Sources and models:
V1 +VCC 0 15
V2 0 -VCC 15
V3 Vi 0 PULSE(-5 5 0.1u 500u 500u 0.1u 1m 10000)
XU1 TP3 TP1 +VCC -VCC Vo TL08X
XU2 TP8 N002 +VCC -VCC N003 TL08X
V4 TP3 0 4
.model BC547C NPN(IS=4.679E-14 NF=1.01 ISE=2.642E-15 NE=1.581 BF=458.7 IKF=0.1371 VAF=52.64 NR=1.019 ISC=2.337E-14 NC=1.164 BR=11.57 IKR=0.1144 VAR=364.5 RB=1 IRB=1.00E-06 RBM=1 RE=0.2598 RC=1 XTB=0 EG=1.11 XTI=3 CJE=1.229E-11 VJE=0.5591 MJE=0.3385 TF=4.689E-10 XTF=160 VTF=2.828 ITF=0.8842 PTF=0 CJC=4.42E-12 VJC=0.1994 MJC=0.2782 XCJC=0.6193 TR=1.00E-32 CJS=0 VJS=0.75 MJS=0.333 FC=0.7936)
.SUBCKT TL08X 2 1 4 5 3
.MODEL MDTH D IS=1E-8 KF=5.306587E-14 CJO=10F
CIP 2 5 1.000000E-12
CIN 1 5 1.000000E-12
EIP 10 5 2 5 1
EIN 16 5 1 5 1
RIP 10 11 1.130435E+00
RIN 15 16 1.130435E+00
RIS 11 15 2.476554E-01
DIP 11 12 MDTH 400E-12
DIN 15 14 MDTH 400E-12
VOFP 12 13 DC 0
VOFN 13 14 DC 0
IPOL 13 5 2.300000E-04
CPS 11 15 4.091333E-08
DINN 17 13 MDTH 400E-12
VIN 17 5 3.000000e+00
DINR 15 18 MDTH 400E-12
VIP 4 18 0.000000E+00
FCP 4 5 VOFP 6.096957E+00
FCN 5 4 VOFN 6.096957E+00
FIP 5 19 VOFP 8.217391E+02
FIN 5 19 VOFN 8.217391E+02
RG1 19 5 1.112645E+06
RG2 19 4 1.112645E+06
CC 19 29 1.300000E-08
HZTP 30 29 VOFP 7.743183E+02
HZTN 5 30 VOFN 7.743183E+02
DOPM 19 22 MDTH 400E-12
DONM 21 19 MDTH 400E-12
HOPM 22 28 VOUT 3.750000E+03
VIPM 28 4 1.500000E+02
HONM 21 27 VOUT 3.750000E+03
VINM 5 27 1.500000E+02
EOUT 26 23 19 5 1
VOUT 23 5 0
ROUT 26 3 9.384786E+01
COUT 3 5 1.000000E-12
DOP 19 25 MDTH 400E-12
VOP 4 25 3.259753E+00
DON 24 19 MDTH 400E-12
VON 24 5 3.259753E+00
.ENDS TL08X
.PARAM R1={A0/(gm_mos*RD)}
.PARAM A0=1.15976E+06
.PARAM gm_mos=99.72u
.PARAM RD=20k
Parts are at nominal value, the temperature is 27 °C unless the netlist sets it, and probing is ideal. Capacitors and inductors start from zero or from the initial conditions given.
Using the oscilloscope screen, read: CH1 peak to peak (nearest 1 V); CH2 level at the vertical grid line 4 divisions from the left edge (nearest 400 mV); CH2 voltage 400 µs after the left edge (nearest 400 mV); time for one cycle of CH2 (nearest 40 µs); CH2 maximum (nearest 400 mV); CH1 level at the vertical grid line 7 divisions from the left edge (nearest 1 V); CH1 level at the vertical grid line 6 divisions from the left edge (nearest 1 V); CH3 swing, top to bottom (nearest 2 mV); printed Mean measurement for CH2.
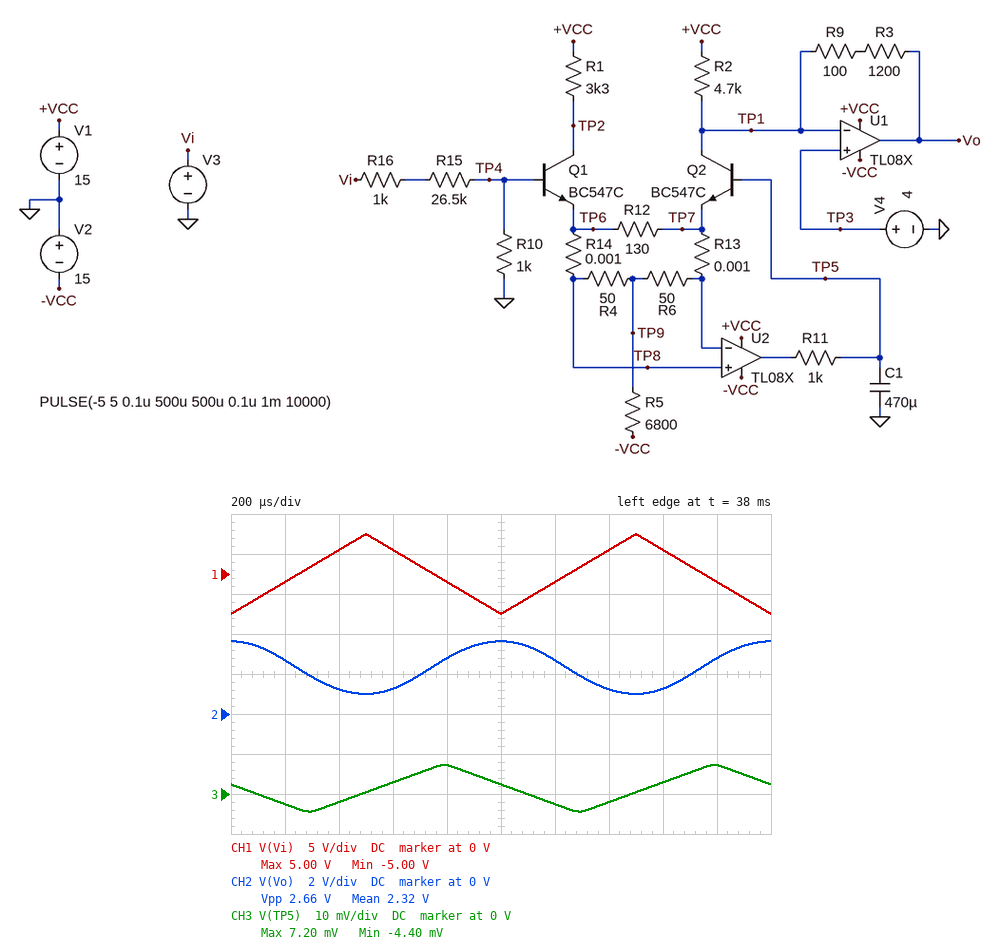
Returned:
10 V
2.8 V
1.2 V
1.00 ms
3.6 V
3 V
-1 V
12 mV
2.32 V
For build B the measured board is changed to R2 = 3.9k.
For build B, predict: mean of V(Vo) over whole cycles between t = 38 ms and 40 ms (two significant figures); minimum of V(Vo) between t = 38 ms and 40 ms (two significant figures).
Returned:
1.7 V
370 mV
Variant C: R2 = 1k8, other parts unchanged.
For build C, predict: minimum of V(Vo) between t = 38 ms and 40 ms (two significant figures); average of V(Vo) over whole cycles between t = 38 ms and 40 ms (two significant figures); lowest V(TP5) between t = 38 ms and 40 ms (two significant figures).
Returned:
-3.9 V
-2.6 V
-4.4 mV
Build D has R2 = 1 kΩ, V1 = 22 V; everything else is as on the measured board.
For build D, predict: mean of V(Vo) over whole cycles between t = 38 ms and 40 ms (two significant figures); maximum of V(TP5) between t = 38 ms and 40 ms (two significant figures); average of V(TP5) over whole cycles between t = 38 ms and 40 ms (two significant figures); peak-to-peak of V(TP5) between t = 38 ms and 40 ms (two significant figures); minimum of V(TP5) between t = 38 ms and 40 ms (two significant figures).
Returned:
-11 V
48 mV
41 mV
14 mV
34 mV
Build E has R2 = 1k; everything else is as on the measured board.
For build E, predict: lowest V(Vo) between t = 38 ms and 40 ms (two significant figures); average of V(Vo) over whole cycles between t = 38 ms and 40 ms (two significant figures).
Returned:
-10 V
-8.9 V
